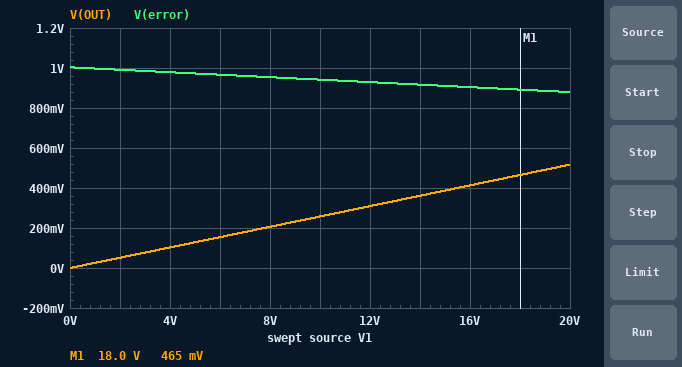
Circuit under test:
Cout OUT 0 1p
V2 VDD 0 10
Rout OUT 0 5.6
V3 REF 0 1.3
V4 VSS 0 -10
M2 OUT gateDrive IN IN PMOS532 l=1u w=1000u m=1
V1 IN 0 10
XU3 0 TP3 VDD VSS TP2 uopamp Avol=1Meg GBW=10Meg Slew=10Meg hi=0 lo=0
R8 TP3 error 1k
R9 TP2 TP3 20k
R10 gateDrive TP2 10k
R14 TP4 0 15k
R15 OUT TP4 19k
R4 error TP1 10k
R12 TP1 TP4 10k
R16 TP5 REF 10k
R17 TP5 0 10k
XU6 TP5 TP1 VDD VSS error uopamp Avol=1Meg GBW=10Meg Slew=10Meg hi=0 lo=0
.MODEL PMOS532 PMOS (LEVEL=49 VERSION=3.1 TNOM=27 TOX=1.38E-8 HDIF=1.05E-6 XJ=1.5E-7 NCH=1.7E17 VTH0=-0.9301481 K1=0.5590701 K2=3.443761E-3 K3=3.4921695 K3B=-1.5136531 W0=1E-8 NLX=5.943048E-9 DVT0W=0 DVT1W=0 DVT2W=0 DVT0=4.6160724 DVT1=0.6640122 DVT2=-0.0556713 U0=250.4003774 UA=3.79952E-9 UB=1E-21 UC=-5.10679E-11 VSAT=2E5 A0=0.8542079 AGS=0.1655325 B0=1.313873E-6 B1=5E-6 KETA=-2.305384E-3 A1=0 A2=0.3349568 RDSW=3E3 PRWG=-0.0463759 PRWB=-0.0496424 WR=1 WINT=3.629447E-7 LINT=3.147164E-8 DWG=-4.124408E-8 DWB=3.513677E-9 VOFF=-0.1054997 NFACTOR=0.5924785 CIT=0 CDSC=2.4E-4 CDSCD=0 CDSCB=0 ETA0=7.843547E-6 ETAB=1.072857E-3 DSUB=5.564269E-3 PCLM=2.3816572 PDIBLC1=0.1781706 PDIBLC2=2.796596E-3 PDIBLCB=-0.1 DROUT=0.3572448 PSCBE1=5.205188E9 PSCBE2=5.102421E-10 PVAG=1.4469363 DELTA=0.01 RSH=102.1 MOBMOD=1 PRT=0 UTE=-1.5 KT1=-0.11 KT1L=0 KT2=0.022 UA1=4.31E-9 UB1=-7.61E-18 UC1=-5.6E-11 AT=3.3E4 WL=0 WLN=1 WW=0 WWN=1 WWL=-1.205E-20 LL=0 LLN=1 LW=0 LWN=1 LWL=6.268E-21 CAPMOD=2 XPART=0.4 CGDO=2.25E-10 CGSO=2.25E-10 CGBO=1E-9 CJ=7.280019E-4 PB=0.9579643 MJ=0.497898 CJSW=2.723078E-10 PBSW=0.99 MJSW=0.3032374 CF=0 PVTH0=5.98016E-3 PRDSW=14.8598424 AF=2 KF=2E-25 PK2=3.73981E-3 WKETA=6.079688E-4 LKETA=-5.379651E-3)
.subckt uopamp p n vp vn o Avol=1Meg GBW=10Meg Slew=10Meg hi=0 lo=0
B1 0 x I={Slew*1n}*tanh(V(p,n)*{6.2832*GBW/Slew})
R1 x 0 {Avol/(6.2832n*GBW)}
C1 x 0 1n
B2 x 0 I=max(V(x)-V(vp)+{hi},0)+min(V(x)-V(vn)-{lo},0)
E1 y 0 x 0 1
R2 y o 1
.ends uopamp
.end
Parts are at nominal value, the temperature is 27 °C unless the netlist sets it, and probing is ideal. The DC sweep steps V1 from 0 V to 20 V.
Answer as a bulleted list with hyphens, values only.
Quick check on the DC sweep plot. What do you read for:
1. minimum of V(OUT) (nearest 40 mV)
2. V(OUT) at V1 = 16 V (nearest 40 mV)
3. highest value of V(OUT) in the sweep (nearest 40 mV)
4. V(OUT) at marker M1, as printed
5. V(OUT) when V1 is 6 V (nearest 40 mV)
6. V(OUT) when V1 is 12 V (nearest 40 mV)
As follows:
- 0 V
- 400 mV
- 520 mV
- 465 mV
- 160 mV
- 320 mV
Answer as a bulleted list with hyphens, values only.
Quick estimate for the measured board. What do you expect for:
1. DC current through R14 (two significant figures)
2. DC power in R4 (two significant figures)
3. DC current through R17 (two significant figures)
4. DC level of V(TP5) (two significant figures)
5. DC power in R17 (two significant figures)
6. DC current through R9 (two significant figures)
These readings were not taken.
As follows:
- 24 µA
- 8.5 µW
- 65 µA
- 650 mV
- 42 µW
- 520 µA
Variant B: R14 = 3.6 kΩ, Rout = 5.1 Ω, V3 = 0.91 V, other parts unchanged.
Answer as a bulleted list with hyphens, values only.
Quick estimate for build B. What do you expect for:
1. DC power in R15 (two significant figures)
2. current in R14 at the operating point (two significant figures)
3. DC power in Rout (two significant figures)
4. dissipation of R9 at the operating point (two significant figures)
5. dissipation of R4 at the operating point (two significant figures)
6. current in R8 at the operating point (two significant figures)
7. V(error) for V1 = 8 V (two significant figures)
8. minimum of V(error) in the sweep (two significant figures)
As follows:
- 530 nW
- 37 µA
- 11 mW
- 5.3 mW
- 10 µW
- 510 µA
- 780 mV
- 750 mV
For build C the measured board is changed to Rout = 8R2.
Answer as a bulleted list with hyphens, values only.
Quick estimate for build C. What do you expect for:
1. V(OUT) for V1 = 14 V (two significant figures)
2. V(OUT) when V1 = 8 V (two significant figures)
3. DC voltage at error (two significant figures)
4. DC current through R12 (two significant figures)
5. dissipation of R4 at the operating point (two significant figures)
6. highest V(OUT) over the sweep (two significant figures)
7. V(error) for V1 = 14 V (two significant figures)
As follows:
- 520 mV
- 300 mV
- 910 mV
- 26 µA
- 7.0 µW
- 750 mV
- 880 mV
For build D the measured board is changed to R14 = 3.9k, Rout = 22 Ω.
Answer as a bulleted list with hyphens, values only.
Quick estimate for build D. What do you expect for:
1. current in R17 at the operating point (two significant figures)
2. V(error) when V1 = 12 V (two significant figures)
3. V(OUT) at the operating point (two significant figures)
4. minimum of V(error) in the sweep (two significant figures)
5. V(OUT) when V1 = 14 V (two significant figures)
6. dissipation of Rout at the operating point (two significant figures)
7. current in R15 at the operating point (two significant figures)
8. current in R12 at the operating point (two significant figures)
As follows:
- 65 µA
- 1.0 V
- 940 mV
- 900 mV
- 1.3 V
- 40 mW
- 35 µA
- 37 µA
